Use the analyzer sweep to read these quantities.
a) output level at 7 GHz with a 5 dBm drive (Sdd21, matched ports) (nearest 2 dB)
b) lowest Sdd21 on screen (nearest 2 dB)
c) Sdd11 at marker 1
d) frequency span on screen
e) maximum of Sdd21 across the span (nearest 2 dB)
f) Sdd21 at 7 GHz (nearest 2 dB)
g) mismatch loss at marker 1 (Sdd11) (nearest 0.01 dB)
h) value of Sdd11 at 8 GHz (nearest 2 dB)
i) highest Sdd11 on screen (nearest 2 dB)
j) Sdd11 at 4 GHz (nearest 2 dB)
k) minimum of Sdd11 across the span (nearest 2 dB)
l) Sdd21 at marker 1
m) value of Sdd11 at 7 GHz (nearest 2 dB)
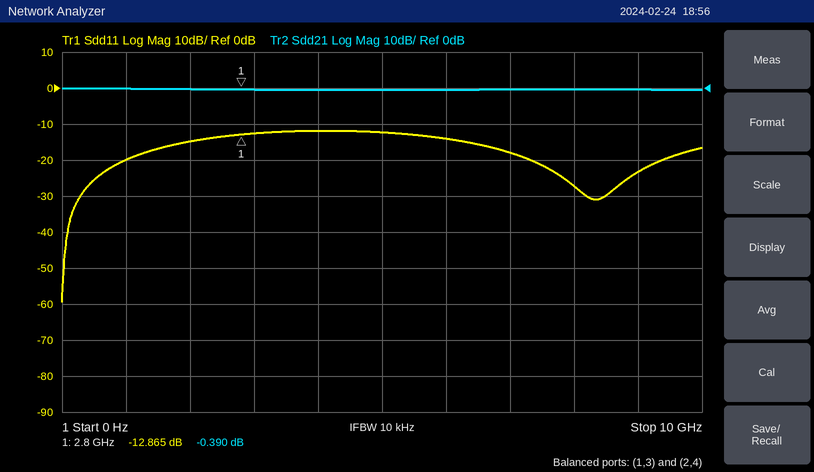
4 dBm
0 dB
-12.865 dB
10 GHz
0 dB
0 dB
0.23 dB
-28 dB
-12 dB
-12 dB
-60 dB
-0.390 dB
-18 dB
